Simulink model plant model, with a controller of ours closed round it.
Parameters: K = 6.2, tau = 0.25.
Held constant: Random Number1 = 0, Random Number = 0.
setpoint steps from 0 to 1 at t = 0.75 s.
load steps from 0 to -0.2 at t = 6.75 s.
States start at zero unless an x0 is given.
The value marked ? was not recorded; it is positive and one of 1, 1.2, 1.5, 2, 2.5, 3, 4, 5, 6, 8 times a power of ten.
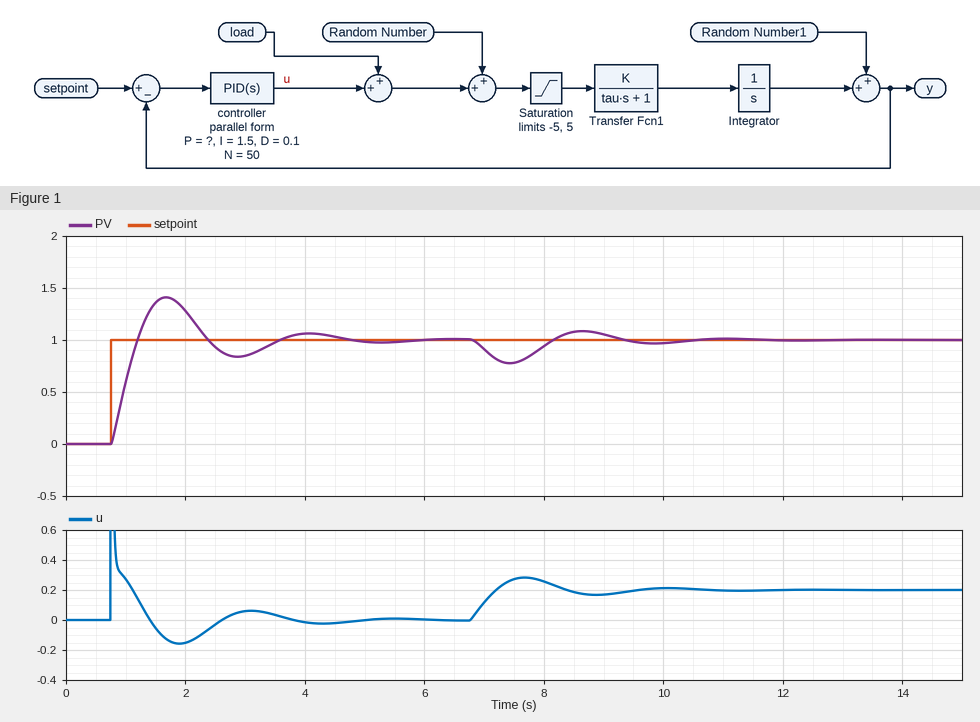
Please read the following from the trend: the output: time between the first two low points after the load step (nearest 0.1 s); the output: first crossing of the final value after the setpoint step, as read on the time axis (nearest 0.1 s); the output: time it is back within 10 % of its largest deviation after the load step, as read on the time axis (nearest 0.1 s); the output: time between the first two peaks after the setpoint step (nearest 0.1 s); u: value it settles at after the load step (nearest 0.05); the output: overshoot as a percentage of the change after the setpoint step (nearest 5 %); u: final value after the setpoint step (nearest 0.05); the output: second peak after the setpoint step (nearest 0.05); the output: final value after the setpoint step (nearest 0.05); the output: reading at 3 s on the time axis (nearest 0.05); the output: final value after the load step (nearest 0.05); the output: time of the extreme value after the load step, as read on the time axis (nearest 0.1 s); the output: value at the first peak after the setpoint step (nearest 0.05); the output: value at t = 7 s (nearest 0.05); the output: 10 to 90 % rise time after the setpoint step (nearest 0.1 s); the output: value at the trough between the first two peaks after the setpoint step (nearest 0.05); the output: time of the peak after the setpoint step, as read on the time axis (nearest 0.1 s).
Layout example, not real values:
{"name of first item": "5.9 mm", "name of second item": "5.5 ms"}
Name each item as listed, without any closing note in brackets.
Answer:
{"the output: time between the first two low points after the load step": "2.4 s", "the output: first crossing of the final value after the setpoint step, as read on the time axis": "1.2 s", "the output: time it is back within 10 % of its largest deviation after the load step, as read on the time axis": "10.2 s", "the output: time between the first two peaks after the setpoint step": "2.4 s", "u: value it settles at after the load step": "0.20", "the output: overshoot as a percentage of the change after the setpoint step": "40 %", "u: final value after the setpoint step": "0.00", "the output: second peak after the setpoint step": "1.05", "the output: final value after the setpoint step": "1.00", "the output: reading at 3 s on the time axis": "0.85", "the output: final value after the load step": "1.00", "the output: time of the extreme value after the load step, as read on the time axis": "7.4 s", "the output: value at the first peak after the setpoint step": "1.40", "the output: value at t = 7 s": "0.90", "the output: 10 to 90 % rise time after the setpoint step": "0.3 s", "the output: value at the trough between the first two peaks after the setpoint step": "0.85", "the output: time of the peak after the setpoint step, as read on the time axis": "1.7 s"}
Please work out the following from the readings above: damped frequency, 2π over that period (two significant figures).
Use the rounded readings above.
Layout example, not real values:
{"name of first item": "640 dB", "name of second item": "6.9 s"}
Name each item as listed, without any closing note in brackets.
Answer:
{"damped frequency, 2π over that period": "2.6 rad/s"}
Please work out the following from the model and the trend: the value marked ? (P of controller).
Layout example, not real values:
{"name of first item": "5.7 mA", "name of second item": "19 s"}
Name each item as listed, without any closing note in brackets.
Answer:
{"the value marked ?": "0.6"}
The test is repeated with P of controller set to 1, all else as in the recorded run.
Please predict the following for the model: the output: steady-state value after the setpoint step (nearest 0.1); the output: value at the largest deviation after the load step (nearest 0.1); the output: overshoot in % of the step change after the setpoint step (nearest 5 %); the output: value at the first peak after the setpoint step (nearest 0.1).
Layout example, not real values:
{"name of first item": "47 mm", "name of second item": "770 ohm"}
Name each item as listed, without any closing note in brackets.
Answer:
{"the output: steady-state value after the setpoint step": "1.0", "the output: value at the largest deviation after the load step": "0.8", "the output: overshoot in % of the step change after the setpoint step": "30 %", "the output: value at the first peak after the setpoint step": "1.3"}
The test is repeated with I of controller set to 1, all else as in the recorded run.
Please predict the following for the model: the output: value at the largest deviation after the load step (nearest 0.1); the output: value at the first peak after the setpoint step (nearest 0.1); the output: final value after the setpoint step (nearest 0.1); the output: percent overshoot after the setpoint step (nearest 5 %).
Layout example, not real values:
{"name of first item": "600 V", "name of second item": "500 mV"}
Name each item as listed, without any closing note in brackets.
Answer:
{"the output: value at the largest deviation after the load step": "0.8", "the output: value at the first peak after the setpoint step": "1.3", "the output: final value after the setpoint step": "1.0", "the output: percent overshoot after the setpoint step": "30 %"}
